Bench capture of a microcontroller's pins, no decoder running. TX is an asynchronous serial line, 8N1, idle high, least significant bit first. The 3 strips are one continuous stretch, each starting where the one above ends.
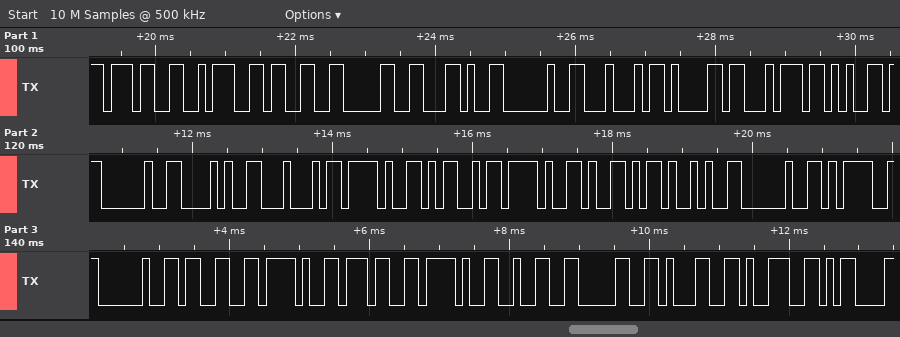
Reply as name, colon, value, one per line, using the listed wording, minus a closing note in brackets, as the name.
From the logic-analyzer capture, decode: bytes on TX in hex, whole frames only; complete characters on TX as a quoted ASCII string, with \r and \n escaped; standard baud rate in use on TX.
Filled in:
bytes on TX in hex, whole frames only: 37 3A 33 30 2C 20 44 61 74 65 20 28 44 2F 4D 2F 59 29 20 3D 20 33 2F 37 2F 32 30 31 39 0D
complete characters on TX as a quoted ASCII string, with \r and \n escaped: "7:30, Date (D/M/Y) = 3/7/2019\r"
standard baud rate in use on TX: 9600 baud
